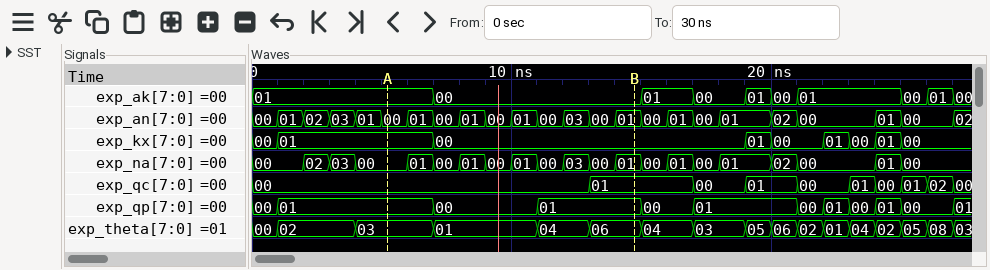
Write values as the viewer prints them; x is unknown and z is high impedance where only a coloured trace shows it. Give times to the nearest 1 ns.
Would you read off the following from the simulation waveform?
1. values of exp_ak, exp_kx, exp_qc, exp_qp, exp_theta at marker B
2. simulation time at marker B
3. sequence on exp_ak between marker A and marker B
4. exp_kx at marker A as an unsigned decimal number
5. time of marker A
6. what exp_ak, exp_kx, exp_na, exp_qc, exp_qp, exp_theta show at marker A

exp_ak=00, exp_kx=00, exp_qc=01, exp_qp=01, exp_theta=06
15 ns
01, 00
1
5 ns
exp_ak=01, exp_kx=01, exp_na=00, exp_qc=00, exp_qp=01, exp_theta=03
